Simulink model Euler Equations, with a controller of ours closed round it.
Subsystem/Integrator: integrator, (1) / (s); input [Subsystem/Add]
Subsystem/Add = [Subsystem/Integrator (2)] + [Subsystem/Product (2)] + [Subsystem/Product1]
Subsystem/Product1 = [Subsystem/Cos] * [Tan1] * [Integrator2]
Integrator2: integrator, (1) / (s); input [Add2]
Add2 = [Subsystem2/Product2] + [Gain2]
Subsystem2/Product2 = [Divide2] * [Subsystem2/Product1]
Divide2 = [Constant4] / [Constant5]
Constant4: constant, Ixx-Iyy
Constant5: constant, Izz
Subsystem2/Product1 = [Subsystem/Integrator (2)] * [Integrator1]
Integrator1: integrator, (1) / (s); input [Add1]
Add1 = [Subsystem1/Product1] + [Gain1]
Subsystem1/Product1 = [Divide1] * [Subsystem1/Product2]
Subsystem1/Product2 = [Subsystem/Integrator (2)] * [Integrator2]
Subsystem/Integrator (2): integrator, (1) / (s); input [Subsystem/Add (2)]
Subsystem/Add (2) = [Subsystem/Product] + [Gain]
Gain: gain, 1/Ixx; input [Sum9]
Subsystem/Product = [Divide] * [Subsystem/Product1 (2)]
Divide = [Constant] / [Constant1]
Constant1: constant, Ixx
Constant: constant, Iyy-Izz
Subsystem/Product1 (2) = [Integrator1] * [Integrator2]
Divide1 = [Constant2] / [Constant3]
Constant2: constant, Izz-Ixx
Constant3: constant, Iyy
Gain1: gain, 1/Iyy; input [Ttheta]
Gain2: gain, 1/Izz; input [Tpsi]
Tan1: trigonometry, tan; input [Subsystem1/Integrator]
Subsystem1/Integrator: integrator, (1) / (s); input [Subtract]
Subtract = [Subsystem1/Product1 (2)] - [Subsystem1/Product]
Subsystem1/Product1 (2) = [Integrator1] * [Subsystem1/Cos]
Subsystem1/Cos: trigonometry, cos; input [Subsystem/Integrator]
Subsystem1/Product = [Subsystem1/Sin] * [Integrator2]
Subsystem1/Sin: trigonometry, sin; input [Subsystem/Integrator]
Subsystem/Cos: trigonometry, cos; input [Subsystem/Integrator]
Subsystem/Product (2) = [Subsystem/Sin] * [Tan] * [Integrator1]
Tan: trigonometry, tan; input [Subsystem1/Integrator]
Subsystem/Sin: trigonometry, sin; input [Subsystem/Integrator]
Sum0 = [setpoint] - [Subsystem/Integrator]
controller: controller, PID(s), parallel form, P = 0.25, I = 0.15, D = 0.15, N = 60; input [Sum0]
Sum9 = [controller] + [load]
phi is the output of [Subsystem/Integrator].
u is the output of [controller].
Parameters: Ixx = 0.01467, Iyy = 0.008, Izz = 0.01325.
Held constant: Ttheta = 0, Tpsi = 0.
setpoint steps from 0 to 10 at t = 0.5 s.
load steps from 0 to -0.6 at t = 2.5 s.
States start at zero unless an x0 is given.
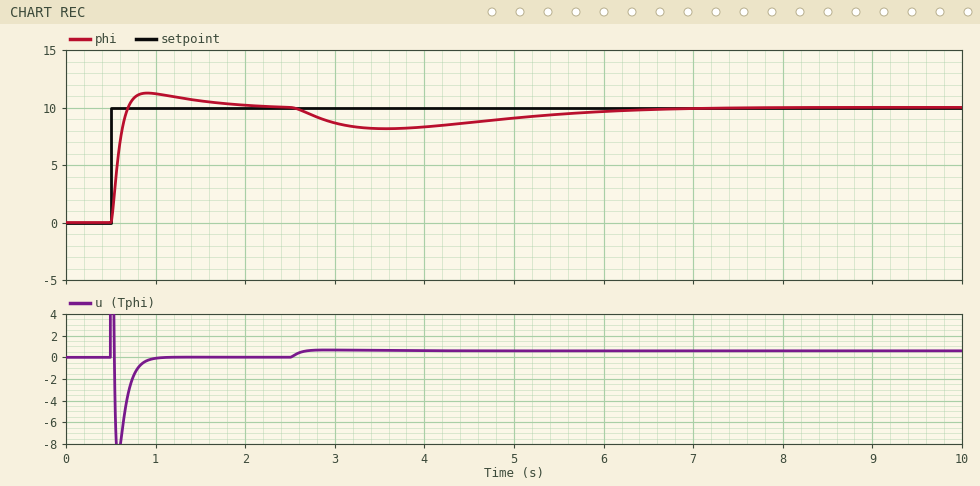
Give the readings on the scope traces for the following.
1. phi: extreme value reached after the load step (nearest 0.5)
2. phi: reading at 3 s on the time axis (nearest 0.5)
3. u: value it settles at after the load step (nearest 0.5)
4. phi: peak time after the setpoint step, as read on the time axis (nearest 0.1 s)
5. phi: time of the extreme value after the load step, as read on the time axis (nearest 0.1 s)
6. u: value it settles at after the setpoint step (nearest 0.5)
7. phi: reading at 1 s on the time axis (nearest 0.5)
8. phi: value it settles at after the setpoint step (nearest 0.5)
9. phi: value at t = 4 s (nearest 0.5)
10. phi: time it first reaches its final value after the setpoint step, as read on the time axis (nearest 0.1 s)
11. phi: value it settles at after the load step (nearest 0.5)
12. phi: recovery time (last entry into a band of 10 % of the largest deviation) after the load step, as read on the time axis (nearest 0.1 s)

8.0
8.5
0.5
0.9 s
3.6 s
0.0
11.0
10.0
8.5
0.7 s
10.0
6.5 s
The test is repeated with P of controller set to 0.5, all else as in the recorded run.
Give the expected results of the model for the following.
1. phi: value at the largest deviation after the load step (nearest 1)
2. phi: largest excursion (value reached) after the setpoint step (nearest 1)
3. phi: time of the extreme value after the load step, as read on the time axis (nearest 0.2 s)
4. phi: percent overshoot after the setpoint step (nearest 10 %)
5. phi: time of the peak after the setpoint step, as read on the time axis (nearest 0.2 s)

9
12
3.2 s
20 %
0.8 s
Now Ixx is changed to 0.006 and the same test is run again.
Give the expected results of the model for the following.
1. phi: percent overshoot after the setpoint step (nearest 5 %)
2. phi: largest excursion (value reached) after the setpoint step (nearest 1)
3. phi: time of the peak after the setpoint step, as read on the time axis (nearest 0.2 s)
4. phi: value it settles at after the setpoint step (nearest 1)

10 %
11
0.6 s
10
